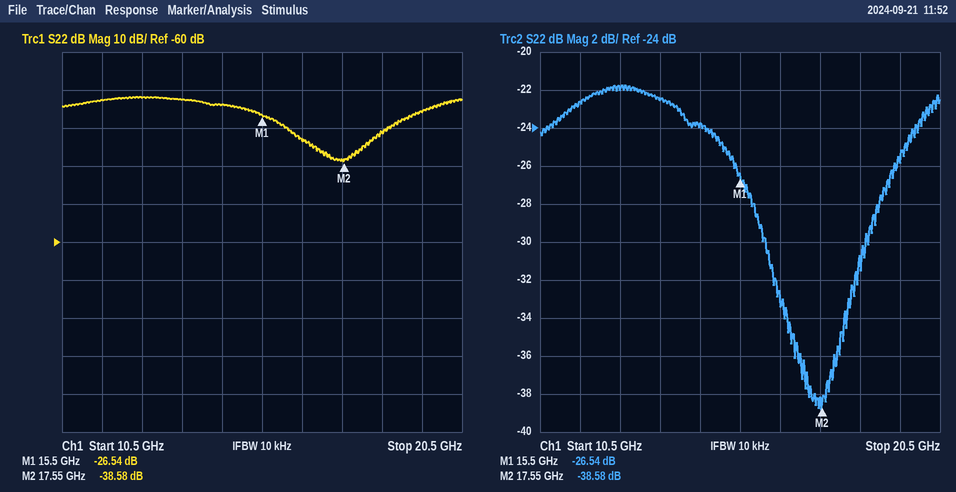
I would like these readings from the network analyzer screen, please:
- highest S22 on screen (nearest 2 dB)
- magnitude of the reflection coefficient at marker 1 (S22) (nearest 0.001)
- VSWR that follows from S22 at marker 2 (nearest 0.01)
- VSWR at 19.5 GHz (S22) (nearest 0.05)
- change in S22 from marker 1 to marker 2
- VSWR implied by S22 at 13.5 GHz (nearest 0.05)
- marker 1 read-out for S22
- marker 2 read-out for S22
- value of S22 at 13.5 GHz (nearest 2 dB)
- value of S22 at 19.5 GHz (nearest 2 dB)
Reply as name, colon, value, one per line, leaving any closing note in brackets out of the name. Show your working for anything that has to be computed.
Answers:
highest S22 on screen: -22 dB
magnitude of the reflection coefficient at marker 1 (S22): 10^(-26.54/20) ≈ 0.047
VSWR that follows from S22 at marker 2: (1 + 0.0118)/(1 − 0.0118) ≈ 1.02
VSWR at 19.5 GHz (S22): |Γ| = 10^(-26/20) = 0.0501; VSWR = (1 + 0.0501)/(1 − 0.0501) ≈ 1.11, so 1.10 to the nearest 0.05
change in S22 from marker 1 to marker 2: -38.58 − (-26.54) = -12.04 dB
VSWR implied by S22 at 13.5 GHz: |Γ| = 10^(-22/20) = 0.0794; VSWR = (1 + 0.0794)/(1 − 0.0794) ≈ 1.17, so 1.15 to the nearest 0.05
marker 1 read-out for S22: -26.54 dB
marker 2 read-out for S22: -38.58 dB
value of S22 at 13.5 GHz: -22 dB
value of S22 at 19.5 GHz: -26 dB
